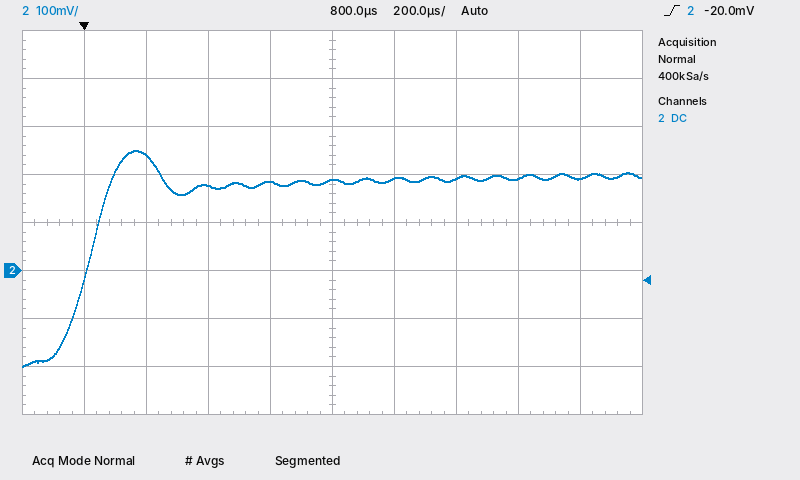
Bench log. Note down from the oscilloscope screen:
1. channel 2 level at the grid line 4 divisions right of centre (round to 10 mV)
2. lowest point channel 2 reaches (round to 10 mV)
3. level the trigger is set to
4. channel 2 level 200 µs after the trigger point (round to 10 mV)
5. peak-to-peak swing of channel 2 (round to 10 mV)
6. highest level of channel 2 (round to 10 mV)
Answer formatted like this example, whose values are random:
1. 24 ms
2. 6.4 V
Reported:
1. 190 mV
2. -200 mV
3. -20.0 mV
4. 240 mV
5. 450 mV
6. 250 mV
